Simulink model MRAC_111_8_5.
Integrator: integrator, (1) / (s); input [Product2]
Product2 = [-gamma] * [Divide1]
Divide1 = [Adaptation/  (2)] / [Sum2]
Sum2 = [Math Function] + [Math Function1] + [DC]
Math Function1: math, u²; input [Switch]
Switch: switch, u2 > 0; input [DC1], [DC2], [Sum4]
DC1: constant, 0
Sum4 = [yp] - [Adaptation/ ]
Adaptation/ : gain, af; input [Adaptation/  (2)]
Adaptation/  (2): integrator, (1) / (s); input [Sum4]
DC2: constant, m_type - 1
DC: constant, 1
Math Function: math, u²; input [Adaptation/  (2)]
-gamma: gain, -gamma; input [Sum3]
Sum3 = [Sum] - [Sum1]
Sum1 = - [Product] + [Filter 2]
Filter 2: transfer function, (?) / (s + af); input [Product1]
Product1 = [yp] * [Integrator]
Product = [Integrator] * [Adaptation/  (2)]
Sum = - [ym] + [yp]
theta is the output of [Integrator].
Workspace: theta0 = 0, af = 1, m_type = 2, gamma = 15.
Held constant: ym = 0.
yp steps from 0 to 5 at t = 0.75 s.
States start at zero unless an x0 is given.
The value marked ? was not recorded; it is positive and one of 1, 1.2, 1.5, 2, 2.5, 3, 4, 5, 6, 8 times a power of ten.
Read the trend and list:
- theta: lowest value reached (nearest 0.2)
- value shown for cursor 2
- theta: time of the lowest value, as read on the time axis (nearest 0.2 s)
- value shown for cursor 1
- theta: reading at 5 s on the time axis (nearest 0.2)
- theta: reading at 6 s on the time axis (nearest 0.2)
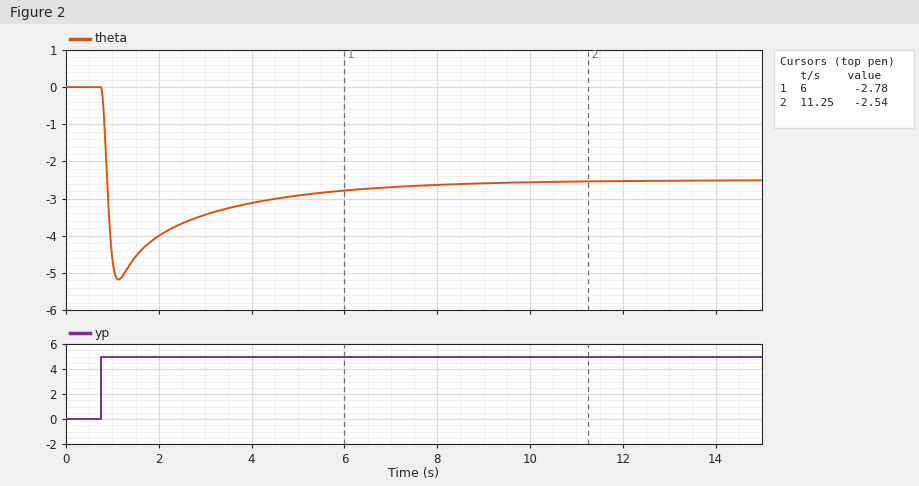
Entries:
-5.2
-2.54
1.2 s
-2.78
-3.0
-2.8
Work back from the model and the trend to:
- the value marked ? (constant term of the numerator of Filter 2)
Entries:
0.6
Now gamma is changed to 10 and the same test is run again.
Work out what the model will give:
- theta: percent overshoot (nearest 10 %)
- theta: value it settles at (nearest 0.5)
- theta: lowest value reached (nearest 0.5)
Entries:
80 %
-2.5
-4.5
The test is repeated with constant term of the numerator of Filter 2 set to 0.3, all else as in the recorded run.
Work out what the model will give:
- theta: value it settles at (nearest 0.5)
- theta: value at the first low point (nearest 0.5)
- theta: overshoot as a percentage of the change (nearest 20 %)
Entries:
-1.5
-4.5
220 %
